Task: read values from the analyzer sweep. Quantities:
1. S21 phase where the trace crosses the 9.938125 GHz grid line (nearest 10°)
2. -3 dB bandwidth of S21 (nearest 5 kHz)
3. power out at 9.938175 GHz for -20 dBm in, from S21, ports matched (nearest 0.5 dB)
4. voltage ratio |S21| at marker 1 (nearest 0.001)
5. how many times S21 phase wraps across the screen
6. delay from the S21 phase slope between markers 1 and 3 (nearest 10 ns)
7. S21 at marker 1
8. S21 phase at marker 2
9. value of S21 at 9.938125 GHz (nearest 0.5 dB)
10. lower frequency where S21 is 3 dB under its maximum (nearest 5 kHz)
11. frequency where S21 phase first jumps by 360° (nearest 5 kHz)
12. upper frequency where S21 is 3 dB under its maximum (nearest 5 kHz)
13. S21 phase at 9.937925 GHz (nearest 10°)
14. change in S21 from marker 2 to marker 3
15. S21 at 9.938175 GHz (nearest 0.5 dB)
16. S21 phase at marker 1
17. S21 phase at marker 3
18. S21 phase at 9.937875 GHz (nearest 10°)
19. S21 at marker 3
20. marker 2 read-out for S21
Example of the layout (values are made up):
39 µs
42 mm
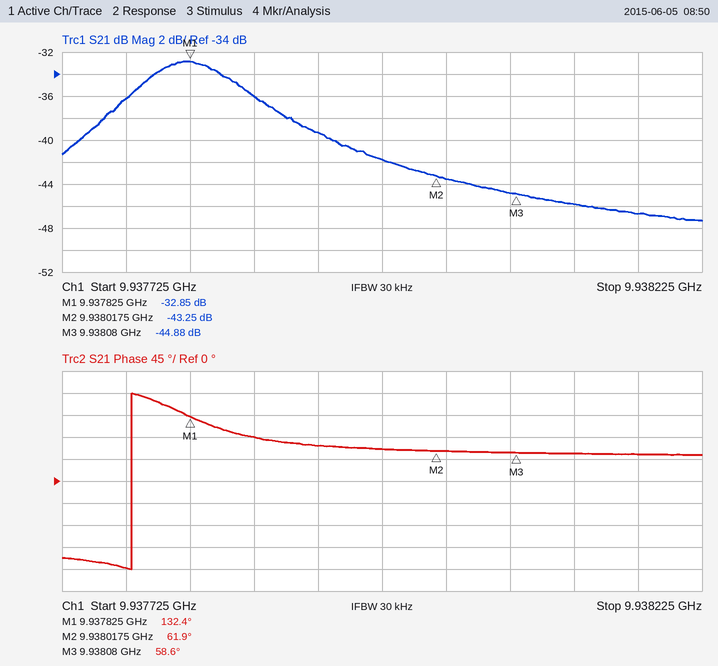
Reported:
60°
95 kHz
-66.5 dBm
0.023
1
800 ns
-32.85 dB
61.9°
-46.0 dB
9.937780 GHz
9.937780 GHz
9.937875 GHz
70°
-1.63 dB
-46.5 dB
132.4°
58.6°
90°
-44.88 dB
-43.25 dB
